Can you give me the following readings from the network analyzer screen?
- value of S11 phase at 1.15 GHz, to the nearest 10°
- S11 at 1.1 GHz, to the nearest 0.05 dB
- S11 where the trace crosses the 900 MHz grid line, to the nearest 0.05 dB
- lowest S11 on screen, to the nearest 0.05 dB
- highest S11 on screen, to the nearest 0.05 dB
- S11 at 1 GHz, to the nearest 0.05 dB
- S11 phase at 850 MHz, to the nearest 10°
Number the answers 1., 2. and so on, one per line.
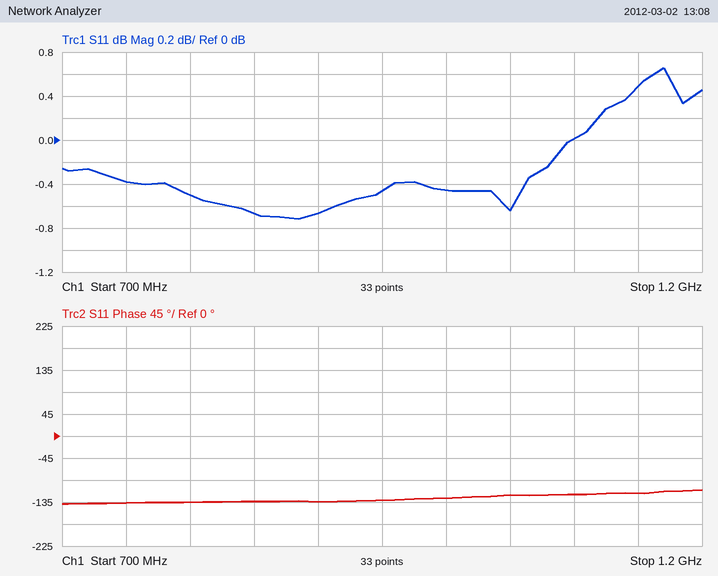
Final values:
1. -120°
2. 0.00 dB
3. -0.65 dB
4. -0.70 dB
5. 0.65 dB
6. -0.45 dB
7. -130°
